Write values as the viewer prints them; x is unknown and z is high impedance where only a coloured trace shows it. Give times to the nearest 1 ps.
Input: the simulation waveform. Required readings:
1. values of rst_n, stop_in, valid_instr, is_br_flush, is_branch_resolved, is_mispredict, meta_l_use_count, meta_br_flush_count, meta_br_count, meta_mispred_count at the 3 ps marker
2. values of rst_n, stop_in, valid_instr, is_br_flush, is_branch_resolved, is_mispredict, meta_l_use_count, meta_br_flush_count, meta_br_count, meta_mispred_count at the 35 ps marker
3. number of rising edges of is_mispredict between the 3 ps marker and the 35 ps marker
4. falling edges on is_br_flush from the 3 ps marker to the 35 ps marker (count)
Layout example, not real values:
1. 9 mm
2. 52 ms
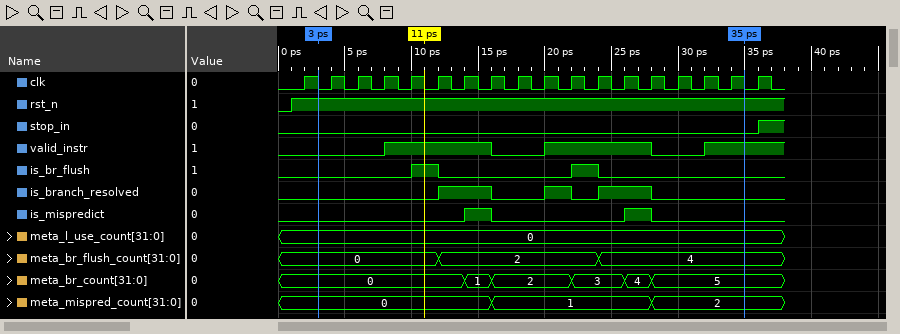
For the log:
1. rst_n=1, stop_in=0, valid_instr=0, is_br_flush=0, is_branch_resolved=0, is_mispredict=0, meta_l_use_count=0, meta_br_flush_count=0, meta_br_count=0, meta_mispred_count=0
2. rst_n=1, stop_in=0, valid_instr=1, is_br_flush=0, is_branch_resolved=0, is_mispredict=0, meta_l_use_count=0, meta_br_flush_count=4, meta_br_count=5, meta_mispred_count=2
3. 2
4. 2
